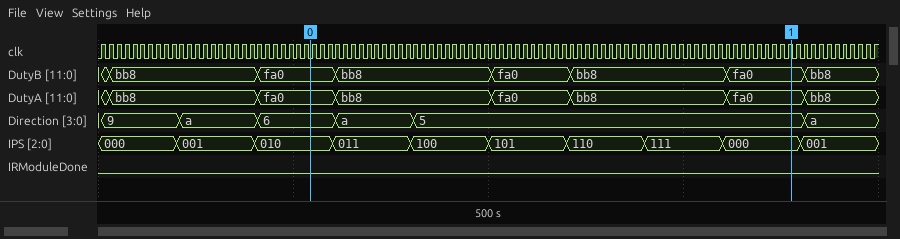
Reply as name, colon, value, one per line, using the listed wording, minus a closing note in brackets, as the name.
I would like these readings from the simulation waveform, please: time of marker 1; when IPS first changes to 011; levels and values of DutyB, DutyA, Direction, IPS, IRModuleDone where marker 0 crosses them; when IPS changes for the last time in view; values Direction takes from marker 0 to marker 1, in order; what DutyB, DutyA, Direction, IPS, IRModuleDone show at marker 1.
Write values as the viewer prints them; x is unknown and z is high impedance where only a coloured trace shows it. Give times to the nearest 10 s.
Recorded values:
time of marker 1: 890 s
when IPS first changes to 011: 300 s
levels and values of DutyB, DutyA, Direction, IPS, IRModuleDone where marker 0 crosses them: DutyB=fa0, DutyA=fa0, Direction=6, IPS=010, IRModuleDone=0
when IPS changes for the last time in view: 900 s
values Direction takes from marker 0 to marker 1, in order: 6, a, 5
what DutyB, DutyA, Direction, IPS, IRModuleDone show at marker 1: DutyB=fa0, DutyA=fa0, Direction=5, IPS=000, IRModuleDone=0
